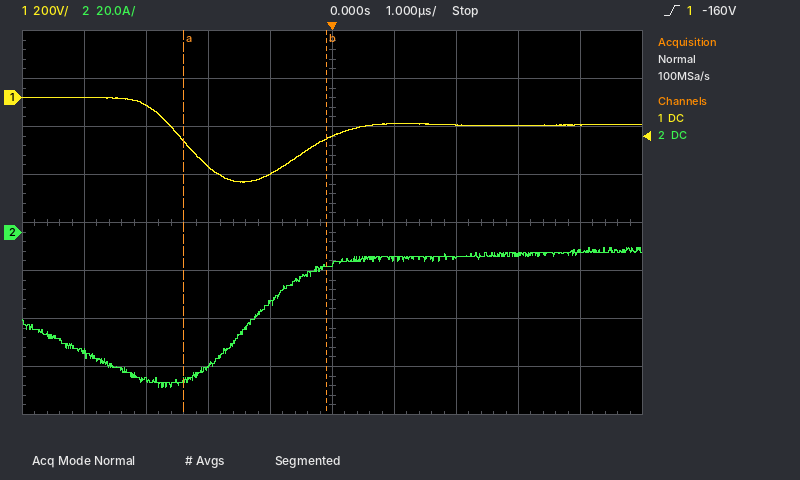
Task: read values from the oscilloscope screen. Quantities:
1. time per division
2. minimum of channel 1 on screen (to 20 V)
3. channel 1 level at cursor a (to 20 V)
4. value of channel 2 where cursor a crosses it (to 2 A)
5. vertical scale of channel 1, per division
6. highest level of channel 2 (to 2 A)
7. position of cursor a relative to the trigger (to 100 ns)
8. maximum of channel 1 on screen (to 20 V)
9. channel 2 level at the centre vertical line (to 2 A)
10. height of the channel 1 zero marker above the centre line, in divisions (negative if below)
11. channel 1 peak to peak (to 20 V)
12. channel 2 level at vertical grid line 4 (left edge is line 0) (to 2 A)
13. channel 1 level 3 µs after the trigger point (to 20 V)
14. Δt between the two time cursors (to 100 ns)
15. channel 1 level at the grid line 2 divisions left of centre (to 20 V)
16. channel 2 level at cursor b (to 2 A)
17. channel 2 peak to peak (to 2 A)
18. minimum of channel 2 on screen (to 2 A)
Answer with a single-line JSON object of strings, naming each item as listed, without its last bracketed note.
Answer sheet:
{"time per division": "1 µs", "minimum of channel 1 on screen": "-360 V", "channel 1 level at cursor a": "-180 V", "value of channel 2 where cursor a crosses it": "-62 A", "vertical scale of channel 1, per division": "200 V", "highest level of channel 2": "-6 A", "position of cursor a relative to the trigger": "-2.4 µs", "maximum of channel 1 on screen": "0 V", "channel 2 level at the centre vertical line": "-14 A", "height of the channel 1 zero marker above the centre line, in divisions": "+2.6 div", "channel 1 peak to peak": "360 V", "channel 2 level at vertical grid line 4 (left edge is line 0)": "-30 A", "channel 1 level 3 µs after the trigger point": "-120 V", "Δt between the two time cursors": "2.3 µs", "channel 1 level at the grid line 2 divisions left of centre": "-280 V", "channel 2 level at cursor b": "-14 A", "channel 2 peak to peak": "58 A", "minimum of channel 2 on screen": "-64 A"}
